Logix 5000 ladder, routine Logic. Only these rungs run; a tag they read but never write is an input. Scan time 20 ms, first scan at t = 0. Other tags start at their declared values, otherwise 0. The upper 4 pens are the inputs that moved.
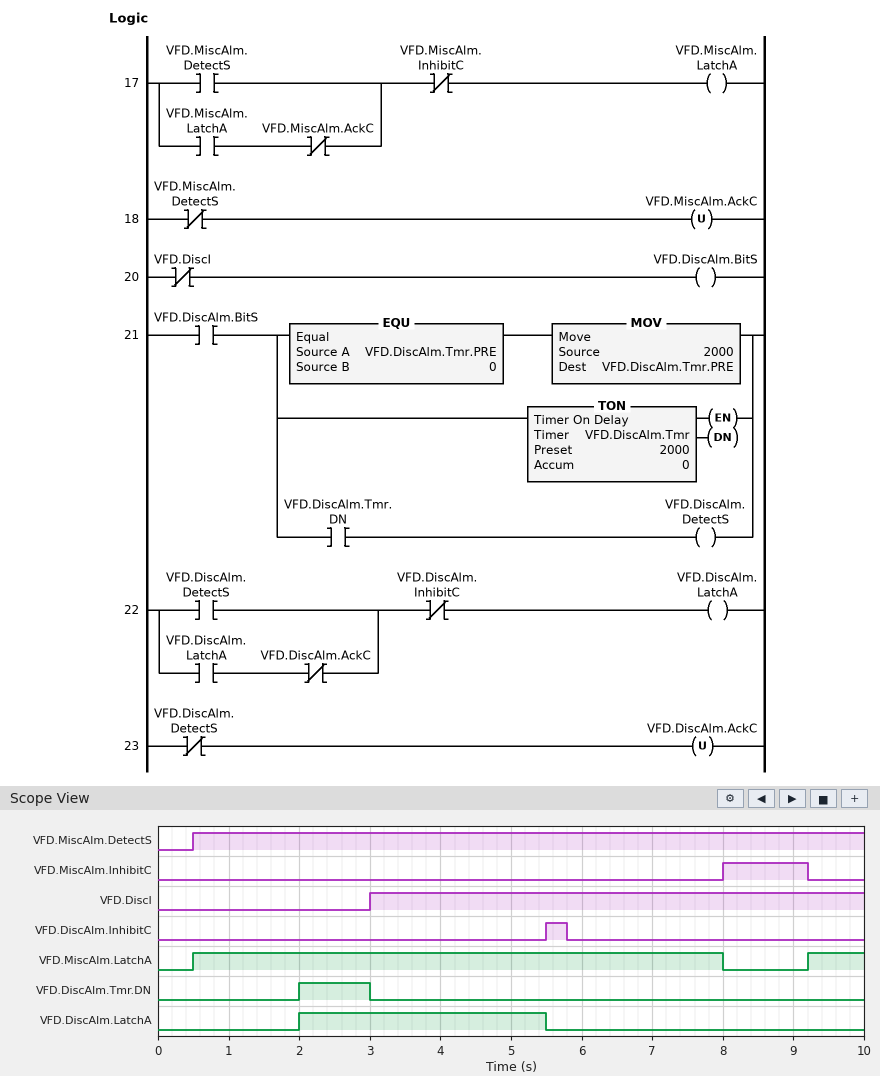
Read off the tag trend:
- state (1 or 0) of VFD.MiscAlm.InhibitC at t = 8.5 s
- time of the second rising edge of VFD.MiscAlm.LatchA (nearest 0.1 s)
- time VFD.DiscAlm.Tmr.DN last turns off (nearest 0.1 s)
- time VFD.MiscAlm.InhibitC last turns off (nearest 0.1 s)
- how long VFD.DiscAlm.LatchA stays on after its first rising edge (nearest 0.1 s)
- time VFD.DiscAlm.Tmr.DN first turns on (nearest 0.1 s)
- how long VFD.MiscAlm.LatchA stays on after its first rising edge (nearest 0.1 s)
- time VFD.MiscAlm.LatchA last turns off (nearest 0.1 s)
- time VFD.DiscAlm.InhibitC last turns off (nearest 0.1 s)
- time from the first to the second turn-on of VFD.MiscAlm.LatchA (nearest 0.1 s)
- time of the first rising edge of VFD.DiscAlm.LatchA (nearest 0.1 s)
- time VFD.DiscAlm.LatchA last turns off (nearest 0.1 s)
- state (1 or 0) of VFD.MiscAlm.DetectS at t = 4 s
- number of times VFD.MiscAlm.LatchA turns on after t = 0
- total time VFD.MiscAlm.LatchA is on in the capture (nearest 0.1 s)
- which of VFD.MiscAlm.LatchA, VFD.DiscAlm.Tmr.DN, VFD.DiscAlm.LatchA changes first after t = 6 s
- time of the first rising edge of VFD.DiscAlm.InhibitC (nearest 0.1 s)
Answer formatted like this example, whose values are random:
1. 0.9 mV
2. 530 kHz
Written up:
1. 1
2. 9.2 s
3. 3.0 s
4. 9.2 s
5. 3.5 s
6. 2.0 s
7. 7.5 s
8. 8.0 s
9. 5.8 s
10. 8.7 s
11. 2.0 s
12. 5.5 s
13. 1
14. 2
15. 8.3 s
16. VFD.MiscAlm.LatchA
17. 5.5 s
